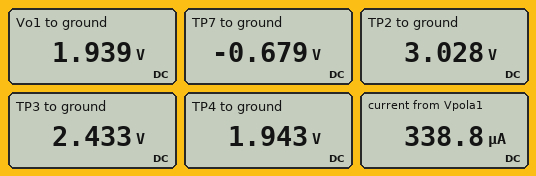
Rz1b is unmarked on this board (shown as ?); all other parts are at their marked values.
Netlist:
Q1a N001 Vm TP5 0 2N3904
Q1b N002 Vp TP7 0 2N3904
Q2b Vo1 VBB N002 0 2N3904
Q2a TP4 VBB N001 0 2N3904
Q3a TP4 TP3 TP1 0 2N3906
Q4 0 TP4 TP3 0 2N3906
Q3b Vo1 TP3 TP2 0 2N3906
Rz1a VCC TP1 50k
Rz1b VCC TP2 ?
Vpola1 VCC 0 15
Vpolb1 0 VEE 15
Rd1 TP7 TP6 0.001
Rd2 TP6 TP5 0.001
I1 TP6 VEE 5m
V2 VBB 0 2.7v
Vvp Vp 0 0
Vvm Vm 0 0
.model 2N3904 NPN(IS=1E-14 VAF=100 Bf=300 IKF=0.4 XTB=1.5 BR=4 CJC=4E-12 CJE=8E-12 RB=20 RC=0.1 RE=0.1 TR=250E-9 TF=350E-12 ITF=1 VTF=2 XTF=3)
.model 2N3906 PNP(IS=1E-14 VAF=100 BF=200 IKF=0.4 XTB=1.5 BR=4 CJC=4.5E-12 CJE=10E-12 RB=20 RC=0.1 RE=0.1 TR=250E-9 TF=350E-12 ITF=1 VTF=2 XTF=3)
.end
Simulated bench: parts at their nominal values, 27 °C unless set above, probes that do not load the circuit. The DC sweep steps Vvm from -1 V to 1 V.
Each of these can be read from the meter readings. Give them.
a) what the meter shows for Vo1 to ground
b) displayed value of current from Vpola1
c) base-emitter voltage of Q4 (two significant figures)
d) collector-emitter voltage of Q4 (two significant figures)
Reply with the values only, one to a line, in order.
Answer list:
1.939 V
338.8 µA
-490 mV
-2.4 V
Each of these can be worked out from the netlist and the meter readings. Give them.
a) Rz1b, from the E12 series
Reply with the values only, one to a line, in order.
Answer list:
120 kΩ
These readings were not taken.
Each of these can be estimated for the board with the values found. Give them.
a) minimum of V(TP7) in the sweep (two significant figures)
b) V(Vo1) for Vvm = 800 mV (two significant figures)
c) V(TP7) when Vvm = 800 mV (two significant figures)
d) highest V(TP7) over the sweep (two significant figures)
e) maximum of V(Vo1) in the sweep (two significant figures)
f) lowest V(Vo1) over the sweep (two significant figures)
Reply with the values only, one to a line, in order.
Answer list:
-700 mV
3.1 V
100 mV
300 mV
3.1 V
1.9 V
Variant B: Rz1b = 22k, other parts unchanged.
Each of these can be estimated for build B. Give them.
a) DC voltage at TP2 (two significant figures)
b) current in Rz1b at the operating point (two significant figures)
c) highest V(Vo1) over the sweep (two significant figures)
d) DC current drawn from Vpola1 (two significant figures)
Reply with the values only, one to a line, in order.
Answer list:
3.1 V
540 µA
3.2 V
780 µA
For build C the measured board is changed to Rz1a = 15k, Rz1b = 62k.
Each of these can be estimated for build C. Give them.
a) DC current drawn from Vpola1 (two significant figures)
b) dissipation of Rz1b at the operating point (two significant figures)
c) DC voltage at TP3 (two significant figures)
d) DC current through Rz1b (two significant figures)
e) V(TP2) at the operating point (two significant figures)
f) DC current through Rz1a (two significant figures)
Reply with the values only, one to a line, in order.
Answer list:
980 µA
2.3 mW
2.5 V
190 µA
3.1 V
790 µA
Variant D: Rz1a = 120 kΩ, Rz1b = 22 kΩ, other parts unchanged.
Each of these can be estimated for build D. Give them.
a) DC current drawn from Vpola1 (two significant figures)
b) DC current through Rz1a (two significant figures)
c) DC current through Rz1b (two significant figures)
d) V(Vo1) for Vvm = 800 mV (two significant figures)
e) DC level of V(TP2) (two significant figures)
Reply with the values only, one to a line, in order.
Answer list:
640 µA
100 µA
540 µA
3.2 V
3.1 V
